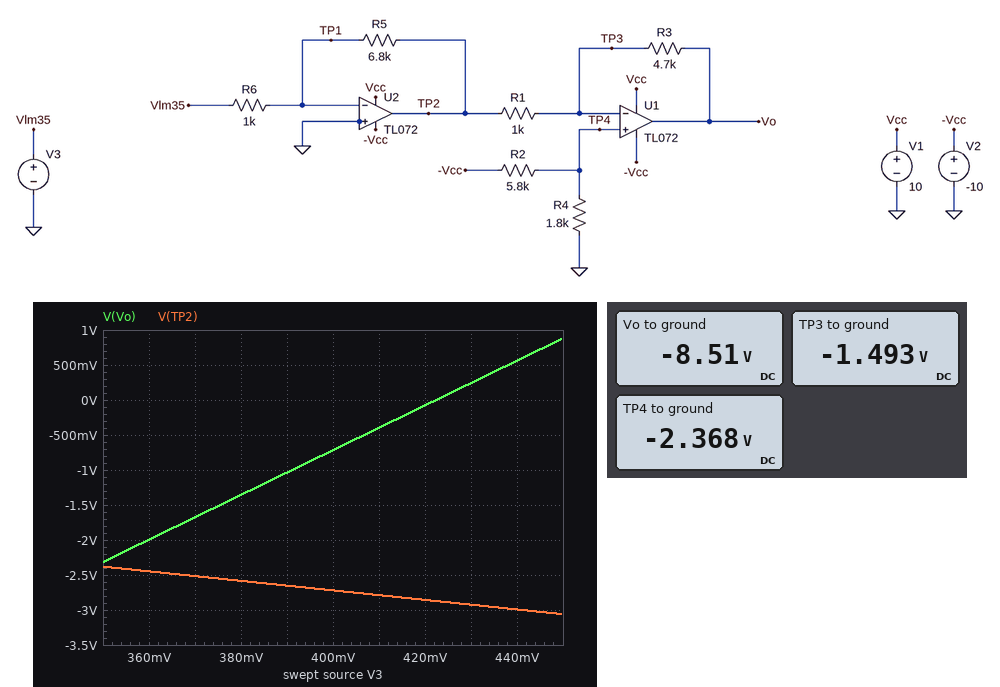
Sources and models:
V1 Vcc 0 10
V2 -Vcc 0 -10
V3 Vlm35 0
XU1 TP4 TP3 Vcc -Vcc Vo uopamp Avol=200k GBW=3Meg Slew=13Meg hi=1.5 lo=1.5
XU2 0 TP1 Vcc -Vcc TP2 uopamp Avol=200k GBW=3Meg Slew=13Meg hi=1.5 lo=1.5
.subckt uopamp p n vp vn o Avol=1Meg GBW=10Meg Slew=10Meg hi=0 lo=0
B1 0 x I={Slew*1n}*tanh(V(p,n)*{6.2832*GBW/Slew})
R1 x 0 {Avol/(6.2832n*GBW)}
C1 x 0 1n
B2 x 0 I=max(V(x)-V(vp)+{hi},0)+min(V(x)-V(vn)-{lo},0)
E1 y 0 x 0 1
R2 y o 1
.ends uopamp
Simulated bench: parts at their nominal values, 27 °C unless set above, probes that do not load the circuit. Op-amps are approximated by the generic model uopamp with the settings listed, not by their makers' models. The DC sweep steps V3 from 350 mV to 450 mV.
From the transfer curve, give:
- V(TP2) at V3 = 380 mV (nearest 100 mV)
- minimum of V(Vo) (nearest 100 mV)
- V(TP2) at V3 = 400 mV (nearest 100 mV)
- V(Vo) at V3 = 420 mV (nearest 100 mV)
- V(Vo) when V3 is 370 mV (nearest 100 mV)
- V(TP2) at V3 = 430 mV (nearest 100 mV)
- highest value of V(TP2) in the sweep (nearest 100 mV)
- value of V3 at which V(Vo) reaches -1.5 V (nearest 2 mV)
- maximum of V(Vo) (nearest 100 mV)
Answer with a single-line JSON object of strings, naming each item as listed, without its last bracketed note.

{"V(TP2) at V3 = 380 mV": "-2.6 V", "minimum of V(Vo)": "-2.3 V", "V(TP2) at V3 = 400 mV": "-2.7 V", "V(Vo) at V3 = 420 mV": "-100 mV", "V(Vo) when V3 is 370 mV": "-1.7 V", "V(TP2) at V3 = 430 mV": "-2.9 V", "highest value of V(TP2) in the sweep": "-2.4 V", "value of V3 at which V(Vo) reaches -1.5 V": "376 mV", "maximum of V(Vo)": "900 mV"}
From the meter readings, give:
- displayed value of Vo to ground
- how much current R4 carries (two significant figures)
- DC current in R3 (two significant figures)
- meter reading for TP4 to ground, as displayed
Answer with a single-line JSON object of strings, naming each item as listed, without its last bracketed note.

{"displayed value of Vo to ground": "-8.51 V", "how much current R4 carries": "1.3 mA", "DC current in R3": "1.5 mA", "meter reading for TP4 to ground, as displayed": "-2.368 V"}
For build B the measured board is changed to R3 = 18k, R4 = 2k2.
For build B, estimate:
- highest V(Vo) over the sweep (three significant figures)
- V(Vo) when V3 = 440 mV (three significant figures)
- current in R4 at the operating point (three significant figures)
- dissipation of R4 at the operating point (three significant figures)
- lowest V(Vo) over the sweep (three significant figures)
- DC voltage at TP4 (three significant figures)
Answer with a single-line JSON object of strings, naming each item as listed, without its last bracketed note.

{"highest V(Vo) over the sweep": "2.83 V", "V(Vo) when V3 = 440 mV": "1.60 V", "current in R4 at the operating point": "1.25 mA", "dissipation of R4 at the operating point": "3.44 mW", "lowest V(Vo) over the sweep": "-8.50 V", "DC voltage at TP4": "-2.75 V"}
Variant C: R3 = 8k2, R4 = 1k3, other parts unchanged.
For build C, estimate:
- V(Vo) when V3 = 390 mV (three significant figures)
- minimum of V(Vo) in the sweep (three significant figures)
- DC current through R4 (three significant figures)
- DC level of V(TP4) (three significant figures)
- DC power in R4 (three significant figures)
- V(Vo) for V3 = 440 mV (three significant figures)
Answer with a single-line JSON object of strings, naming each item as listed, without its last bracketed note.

{"V(Vo) when V3 = 390 mV": "4.90 V", "minimum of V(Vo) in the sweep": "2.67 V", "DC current through R4": "1.41 mA", "DC level of V(TP4)": "-1.83 V", "DC power in R4": "2.58 mW", "V(Vo) for V3 = 440 mV": "7.69 V"}
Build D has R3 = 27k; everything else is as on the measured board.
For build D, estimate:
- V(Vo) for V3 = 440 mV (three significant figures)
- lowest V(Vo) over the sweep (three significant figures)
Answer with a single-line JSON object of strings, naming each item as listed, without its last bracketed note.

{"V(Vo) for V3 = 440 mV": "8.50 V", "lowest V(Vo) over the sweep": "-2.06 V"}
